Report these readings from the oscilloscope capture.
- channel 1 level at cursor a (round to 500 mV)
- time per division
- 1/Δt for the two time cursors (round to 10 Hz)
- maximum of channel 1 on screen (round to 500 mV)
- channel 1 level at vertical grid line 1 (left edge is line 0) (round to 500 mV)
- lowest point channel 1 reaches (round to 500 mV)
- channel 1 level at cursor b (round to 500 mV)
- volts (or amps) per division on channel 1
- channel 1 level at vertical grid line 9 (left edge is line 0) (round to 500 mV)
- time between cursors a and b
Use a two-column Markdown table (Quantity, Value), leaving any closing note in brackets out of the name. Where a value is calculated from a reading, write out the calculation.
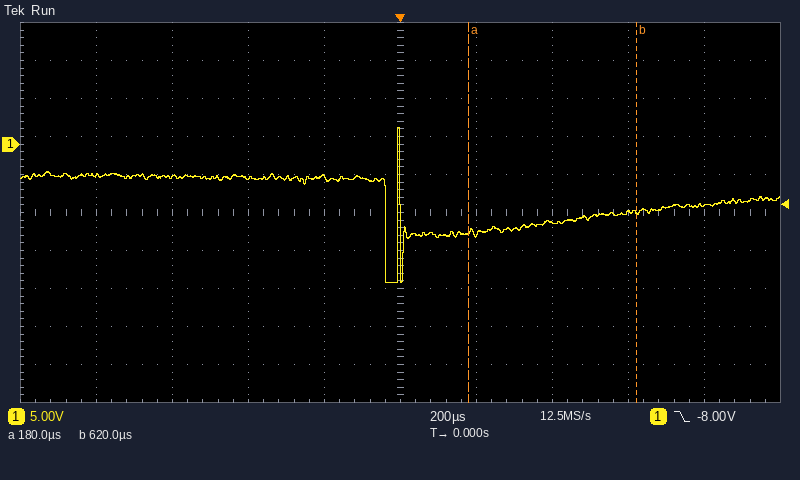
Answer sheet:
| Quantity | Value |
|---|---|
| channel 1 level at cursor a | -11.5 V |
| time per division | 200 µs |
| 1/Δt for the two time cursors | 1 / 440 µs ≈ 2.27 kHz |
| maximum of channel 1 on screen | 2.0 V |
| channel 1 level at vertical grid line 1 (left edge is line 0) | -4.0 V |
| lowest point channel 1 reaches | -18.0 V |
| channel 1 level at cursor b | -9.0 V |
| volts (or amps) per division on channel 1 | 5 V |
| channel 1 level at vertical grid line 9 (left edge is line 0) | -8.0 V |
| time between cursors a and b | 620 µs − (180 µs) = 440 µs |
